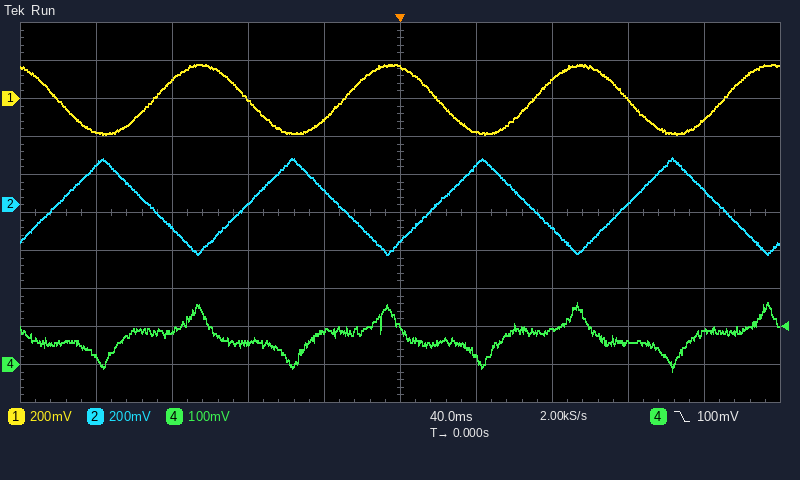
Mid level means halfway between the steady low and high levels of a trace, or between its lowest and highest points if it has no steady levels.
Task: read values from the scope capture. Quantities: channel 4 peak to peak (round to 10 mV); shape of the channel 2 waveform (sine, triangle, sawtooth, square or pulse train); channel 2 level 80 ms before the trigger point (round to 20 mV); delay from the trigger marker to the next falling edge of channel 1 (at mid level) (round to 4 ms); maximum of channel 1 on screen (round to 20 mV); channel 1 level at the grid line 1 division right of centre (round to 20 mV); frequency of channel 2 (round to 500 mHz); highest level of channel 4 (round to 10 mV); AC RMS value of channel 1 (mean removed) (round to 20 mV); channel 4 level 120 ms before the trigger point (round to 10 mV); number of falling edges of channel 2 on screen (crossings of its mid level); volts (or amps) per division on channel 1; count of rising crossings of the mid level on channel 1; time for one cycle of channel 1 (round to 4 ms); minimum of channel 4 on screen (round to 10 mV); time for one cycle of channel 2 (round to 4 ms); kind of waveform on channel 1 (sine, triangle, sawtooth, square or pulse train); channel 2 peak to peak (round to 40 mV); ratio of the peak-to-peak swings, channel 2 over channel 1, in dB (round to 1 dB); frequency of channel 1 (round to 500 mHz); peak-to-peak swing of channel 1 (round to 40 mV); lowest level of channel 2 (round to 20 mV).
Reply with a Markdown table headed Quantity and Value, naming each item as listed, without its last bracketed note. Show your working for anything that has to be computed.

| Quantity | Value |
|---|---|
| channel 4 peak to peak | 160 mV − (-20 mV) = 180 mV |
| shape of the channel 2 waveform | triangle |
| channel 2 level 80 ms before the trigger point | 0 mV |
| delay from the trigger marker to the next falling edge of channel 1 (at mid level) | 20 ms |
| maximum of channel 1 on screen | 180 mV |
| channel 1 level at the grid line 1 division right of centre | -180 mV |
| frequency of channel 2 | 1 / 100 ms ≈ 10.0 Hz |
| highest level of channel 4 | 160 mV |
| AC RMS value of channel 1 (mean removed) | 360 mV / (2√2) ≈ 127 mV, so 120 mV to the nearest 20 mV |
| channel 4 level 120 ms before the trigger point | 90 mV |
| number of falling edges of channel 2 on screen | 4 |
| volts (or amps) per division on channel 1 | 200 mV |
| count of rising crossings of the mid level on channel 1 | 4 |
| time for one cycle of channel 1 | 100 ms |
| minimum of channel 4 on screen | -20 mV |
| time for one cycle of channel 2 | 100 ms |
| kind of waveform on channel 1 | sine |
| channel 2 peak to peak | 520 mV |
| ratio of the peak-to-peak swings, channel 2 over channel 1, in dB | 20 log10(520 mV / 360 mV) ≈ 3 dB |
| frequency of channel 1 | 1 / 100 ms ≈ 10.0 Hz |
| peak-to-peak swing of channel 1 | 360 mV |
| lowest level of channel 2 | -260 mV |
